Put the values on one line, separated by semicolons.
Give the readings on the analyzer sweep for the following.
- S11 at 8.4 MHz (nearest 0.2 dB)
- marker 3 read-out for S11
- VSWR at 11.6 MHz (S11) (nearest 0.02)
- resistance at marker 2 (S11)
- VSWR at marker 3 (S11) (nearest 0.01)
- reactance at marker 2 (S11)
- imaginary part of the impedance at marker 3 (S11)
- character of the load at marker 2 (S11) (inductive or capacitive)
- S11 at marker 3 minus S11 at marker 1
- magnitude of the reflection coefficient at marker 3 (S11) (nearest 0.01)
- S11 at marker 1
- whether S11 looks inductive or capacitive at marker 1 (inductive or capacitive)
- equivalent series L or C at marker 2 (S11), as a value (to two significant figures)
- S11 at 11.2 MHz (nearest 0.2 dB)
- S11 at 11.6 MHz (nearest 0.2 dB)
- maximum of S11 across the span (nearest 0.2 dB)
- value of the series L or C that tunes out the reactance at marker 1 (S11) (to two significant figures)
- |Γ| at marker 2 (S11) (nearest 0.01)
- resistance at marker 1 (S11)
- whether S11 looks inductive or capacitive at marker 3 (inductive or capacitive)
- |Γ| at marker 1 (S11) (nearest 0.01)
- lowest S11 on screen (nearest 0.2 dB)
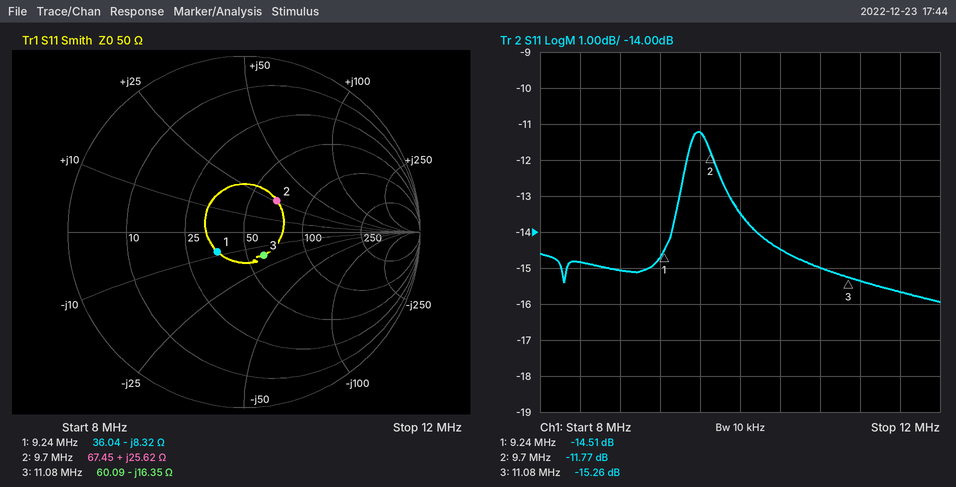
-14.8 dB; -15.26 dB; 1.40; 67.45 Ω; 1.42; +25.62 Ω; -16.35 Ω; inductive; -0.75 dB; 0.17; -14.51 dB; capacitive; 420 nH; -15.4 dB; -15.6 dB; -11.2 dB; 140 nH; 0.26; 36.04 Ω; capacitive; 0.19; -16.0 dB
